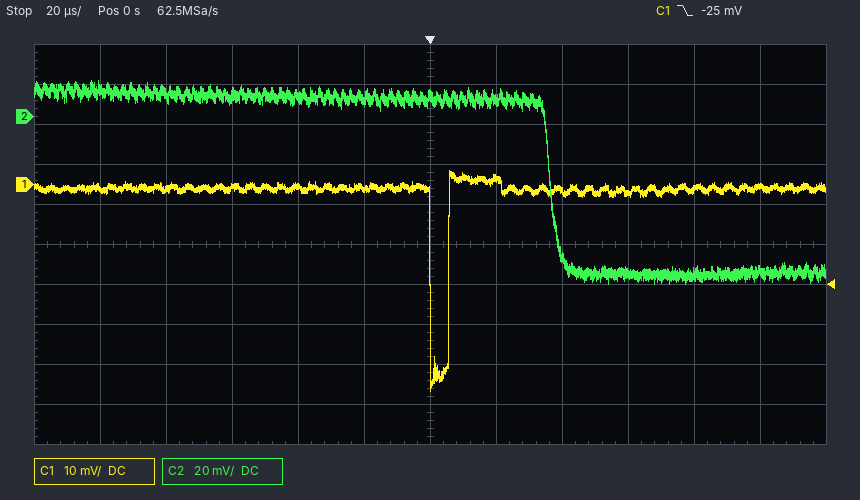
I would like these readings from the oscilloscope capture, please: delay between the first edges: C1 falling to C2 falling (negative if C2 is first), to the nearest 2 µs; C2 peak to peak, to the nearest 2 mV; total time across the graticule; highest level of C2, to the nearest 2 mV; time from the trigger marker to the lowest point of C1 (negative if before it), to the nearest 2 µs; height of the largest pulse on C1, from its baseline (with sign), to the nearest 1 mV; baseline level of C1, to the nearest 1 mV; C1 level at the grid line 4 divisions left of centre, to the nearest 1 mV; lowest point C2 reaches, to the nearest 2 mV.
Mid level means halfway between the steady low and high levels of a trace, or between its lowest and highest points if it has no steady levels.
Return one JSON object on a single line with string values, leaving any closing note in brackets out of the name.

{"delay between the first edges: C1 falling to C2 falling (negative if C2 is first), to the nearest 2 µs": "+36 µs", "C2 peak to peak, to the nearest 2 mV": "102 mV", "total time across the graticule": "240 µs", "highest level of C2, to the nearest 2 mV": "18 mV", "time from the trigger marker to the lowest point of C1 (negative if before it), to the nearest 2 µs": "0 µs", "height of the largest pulse on C1, from its baseline (with sign), to the nearest 1 mV": "-51 mV", "baseline level of C1, to the nearest 1 mV": "-1 mV", "C1 level at the grid line 4 divisions left of centre, to the nearest 1 mV": "-1 mV", "lowest point C2 reaches, to the nearest 2 mV": "-84 mV"}
